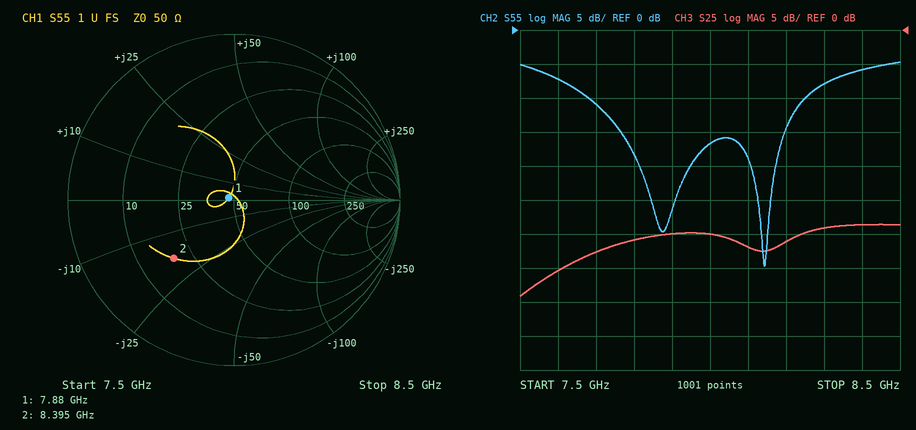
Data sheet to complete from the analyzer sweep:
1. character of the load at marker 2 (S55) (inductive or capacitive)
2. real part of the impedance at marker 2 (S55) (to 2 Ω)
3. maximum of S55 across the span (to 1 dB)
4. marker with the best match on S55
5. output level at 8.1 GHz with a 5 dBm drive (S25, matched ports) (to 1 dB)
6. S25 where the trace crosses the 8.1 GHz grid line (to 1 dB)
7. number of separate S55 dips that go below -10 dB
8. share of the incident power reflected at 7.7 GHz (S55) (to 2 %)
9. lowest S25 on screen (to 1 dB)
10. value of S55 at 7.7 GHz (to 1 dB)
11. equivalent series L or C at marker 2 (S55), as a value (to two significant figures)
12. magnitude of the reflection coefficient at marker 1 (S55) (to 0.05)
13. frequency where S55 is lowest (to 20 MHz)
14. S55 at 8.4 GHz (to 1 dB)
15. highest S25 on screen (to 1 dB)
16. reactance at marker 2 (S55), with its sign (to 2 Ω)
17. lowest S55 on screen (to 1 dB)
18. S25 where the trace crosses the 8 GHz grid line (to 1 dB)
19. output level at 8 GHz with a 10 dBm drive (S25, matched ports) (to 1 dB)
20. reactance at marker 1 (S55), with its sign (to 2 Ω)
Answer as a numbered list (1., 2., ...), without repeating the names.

1. capacitive
2. 18 Ω
3. -5 dB
4. marker 1
5. -27 dBm
6. -32 dB
7. 2
8. 8 %
9. -39 dB
10. -11 dB
11. 1.1 pF
12. 0.05
13. 8.14 GHz
14. -6 dB
15. -29 dB
16. -18 Ω
17. -35 dB
18. -30 dB
19. -20 dBm
20. +2 Ω
